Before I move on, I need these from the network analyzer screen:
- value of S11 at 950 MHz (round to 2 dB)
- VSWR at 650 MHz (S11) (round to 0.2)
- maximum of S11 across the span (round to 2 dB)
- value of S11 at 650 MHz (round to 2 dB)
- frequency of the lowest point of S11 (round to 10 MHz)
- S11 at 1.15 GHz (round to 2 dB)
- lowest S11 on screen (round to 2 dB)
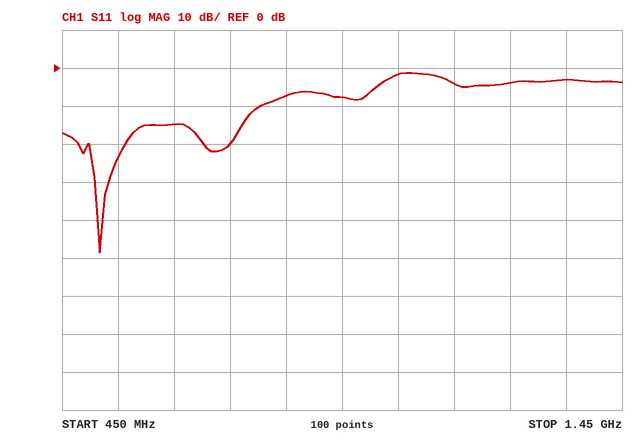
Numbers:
-8 dB
1.4
-2 dB
-14 dB
520 MHz
-4 dB
-48 dB
